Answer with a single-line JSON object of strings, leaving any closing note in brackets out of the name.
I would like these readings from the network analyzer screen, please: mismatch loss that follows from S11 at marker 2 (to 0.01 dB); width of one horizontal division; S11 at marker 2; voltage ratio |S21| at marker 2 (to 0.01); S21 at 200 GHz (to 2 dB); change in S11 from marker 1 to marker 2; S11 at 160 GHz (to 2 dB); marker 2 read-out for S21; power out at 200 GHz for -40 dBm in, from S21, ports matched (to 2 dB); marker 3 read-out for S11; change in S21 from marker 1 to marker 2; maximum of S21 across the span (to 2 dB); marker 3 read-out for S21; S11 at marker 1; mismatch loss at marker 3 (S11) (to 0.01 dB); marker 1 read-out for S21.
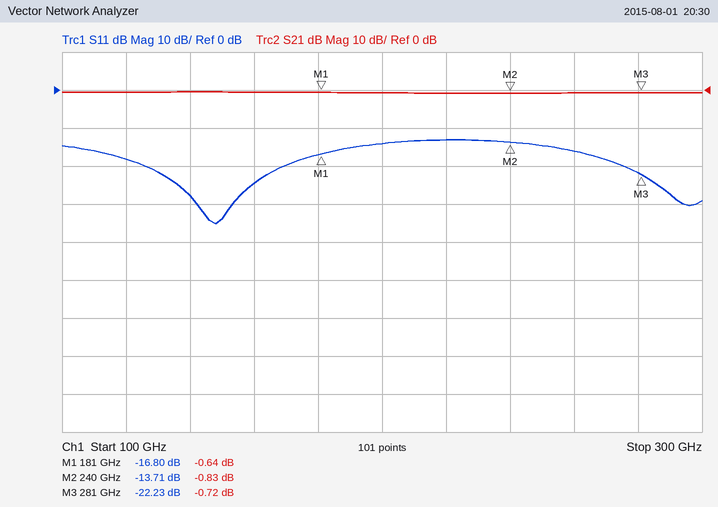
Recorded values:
{"mismatch loss that follows from S11 at marker 2": "0.19 dB", "width of one horizontal division": "20 GHz", "S11 at marker 2": "-13.71 dB", "voltage ratio |S21| at marker 2": "0.91", "S21 at 200 GHz": "0 dB", "change in S11 from marker 1 to marker 2": "3.09 dB", "S11 at 160 GHz": "-24 dB", "marker 2 read-out for S21": "-0.83 dB", "power out at 200 GHz for -40 dBm in, from S21, ports matched": "-40 dBm", "marker 3 read-out for S11": "-22.23 dB", "change in S21 from marker 1 to marker 2": "-0.19 dB", "maximum of S21 across the span": "0 dB", "marker 3 read-out for S21": "-0.72 dB", "S11 at marker 1": "-16.80 dB", "mismatch loss at marker 3 (S11)": "0.03 dB", "marker 1 read-out for S21": "-0.64 dB"}
